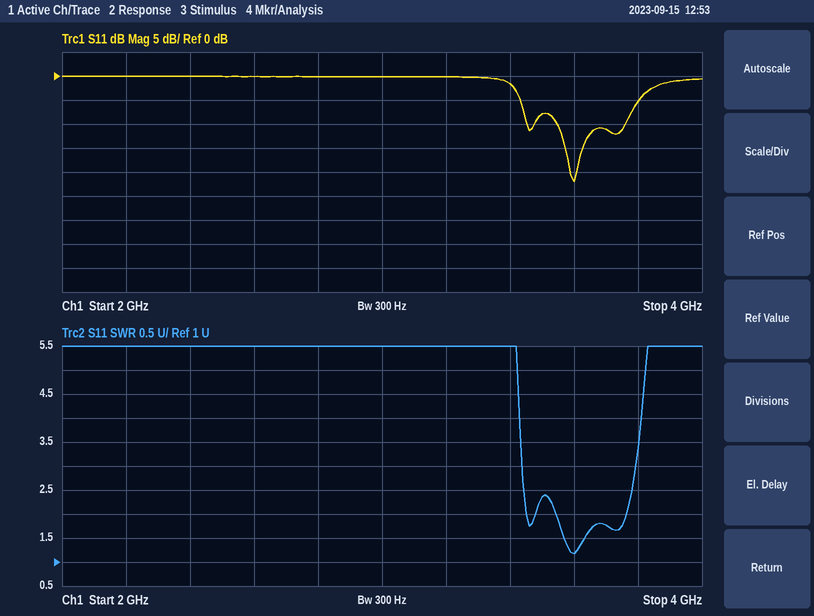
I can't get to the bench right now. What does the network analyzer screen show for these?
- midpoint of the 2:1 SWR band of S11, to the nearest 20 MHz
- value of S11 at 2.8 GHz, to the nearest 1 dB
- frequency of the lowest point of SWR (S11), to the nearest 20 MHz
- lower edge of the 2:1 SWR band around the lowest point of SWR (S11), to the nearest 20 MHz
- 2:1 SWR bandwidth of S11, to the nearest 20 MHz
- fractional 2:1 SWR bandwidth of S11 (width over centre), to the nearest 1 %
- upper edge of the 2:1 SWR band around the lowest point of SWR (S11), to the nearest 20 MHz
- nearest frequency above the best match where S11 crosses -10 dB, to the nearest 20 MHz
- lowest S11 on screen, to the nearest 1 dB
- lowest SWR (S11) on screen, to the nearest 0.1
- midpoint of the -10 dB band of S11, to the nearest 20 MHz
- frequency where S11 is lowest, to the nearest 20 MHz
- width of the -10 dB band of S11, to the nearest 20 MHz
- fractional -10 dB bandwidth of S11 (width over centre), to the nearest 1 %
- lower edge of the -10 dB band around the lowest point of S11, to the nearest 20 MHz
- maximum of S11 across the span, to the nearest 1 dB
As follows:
3.66 GHz
0 dB
3.60 GHz
3.54 GHz
220 MHz
6 %
3.76 GHz
3.76 GHz
-22 dB
1.2
3.66 GHz
3.60 GHz
220 MHz
6 %
3.54 GHz
0 dB
